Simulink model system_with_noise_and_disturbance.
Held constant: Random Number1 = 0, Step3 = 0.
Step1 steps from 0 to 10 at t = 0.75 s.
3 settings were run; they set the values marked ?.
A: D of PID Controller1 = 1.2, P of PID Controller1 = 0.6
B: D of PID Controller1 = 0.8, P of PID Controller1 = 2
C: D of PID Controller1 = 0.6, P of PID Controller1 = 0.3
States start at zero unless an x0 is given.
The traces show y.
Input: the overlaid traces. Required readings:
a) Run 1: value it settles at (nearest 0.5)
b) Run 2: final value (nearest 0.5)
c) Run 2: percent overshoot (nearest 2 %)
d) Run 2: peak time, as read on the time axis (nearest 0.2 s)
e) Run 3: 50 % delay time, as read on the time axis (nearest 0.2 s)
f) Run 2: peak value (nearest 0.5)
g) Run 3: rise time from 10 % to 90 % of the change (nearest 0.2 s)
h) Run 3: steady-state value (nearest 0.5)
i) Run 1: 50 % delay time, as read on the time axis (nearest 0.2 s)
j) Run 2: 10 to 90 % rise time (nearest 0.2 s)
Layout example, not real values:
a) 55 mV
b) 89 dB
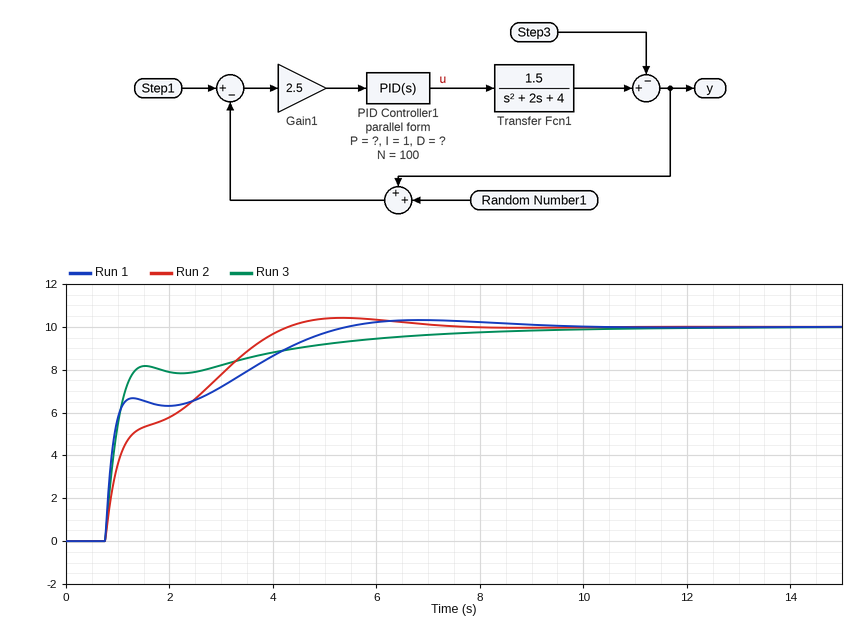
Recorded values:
a) 10.0
b) 10.0
c) 4 %
d) 5.4 s
e) 1.0 s
f) 10.5
g) 3.6 s
h) 10.0
i) 1.0 s
j) 2.8 s
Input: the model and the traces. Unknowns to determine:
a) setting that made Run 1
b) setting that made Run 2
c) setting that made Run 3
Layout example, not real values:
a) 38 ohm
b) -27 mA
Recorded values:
a) A
b) C
c) B
